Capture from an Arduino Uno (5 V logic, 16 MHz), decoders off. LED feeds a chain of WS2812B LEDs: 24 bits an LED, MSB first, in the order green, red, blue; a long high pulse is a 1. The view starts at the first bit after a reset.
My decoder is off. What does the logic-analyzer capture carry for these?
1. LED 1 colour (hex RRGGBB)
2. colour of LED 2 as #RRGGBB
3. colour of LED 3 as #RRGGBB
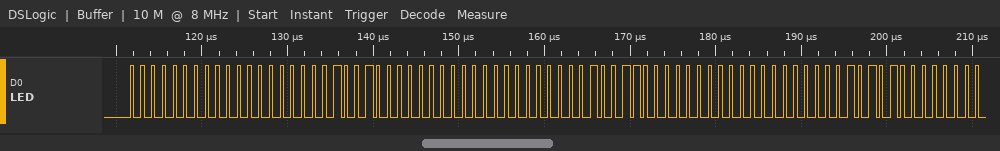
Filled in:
#000012
#000013
#000015
